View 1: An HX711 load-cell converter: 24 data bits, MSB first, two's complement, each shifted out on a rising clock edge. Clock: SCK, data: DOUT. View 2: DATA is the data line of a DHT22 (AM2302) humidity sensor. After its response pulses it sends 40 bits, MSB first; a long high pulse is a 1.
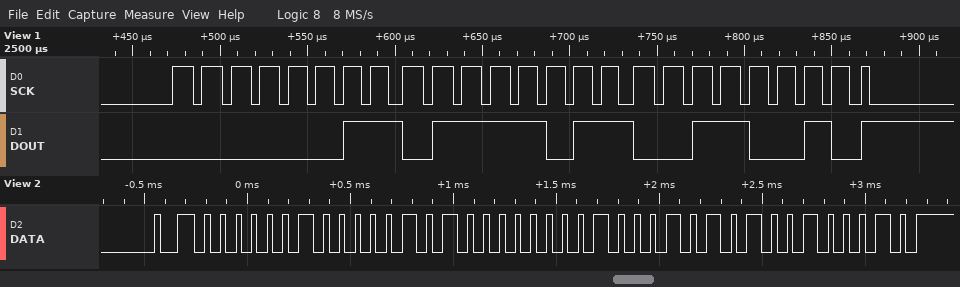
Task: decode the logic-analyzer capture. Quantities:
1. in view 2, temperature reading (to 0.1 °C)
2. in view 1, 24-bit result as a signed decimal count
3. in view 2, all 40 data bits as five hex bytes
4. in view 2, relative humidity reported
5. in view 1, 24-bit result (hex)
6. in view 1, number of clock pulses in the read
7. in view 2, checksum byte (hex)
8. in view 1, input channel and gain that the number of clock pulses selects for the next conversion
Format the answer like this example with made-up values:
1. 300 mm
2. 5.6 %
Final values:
1. 27.7 °C
2. 228146
3. 02 0A 01 15 22
4. 52.2 %
5. 0x037B32
6. 25
7. 0x22
8. channel A, gain 128
